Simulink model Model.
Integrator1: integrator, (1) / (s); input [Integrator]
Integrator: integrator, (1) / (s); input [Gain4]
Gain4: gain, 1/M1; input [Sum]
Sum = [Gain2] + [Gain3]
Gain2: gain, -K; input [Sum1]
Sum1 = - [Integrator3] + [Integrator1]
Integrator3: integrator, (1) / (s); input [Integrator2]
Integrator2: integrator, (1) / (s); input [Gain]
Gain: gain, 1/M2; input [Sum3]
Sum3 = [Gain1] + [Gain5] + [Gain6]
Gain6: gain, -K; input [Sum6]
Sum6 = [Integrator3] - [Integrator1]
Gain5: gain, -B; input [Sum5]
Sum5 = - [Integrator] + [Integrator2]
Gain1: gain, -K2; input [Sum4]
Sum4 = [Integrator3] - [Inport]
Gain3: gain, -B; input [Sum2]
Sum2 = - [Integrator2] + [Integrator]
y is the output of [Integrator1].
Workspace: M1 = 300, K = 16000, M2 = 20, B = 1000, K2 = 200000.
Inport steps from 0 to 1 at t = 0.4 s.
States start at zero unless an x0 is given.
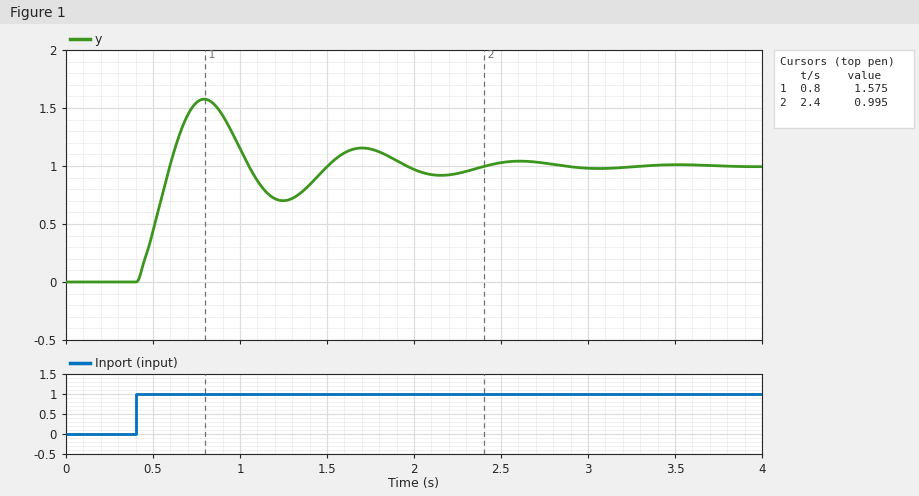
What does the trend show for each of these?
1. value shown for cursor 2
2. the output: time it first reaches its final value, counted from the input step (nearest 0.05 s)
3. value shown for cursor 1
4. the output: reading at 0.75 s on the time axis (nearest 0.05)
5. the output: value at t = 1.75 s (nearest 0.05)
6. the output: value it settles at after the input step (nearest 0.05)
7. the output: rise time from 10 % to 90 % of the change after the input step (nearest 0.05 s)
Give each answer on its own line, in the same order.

0.995
0.20 s
1.575
1.55
1.15
1.00
0.15 s
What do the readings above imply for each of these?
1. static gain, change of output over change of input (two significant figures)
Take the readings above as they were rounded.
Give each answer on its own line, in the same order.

1.0
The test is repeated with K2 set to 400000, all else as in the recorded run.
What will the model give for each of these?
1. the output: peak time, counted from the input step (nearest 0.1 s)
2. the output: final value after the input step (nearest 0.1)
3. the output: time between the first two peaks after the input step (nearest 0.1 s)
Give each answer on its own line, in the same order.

0.4 s
1.0
0.9 s
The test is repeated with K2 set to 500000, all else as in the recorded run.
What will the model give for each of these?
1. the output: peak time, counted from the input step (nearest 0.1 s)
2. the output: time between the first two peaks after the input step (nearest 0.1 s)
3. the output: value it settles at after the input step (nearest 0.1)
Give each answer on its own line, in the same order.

0.4 s
0.9 s
1.0
